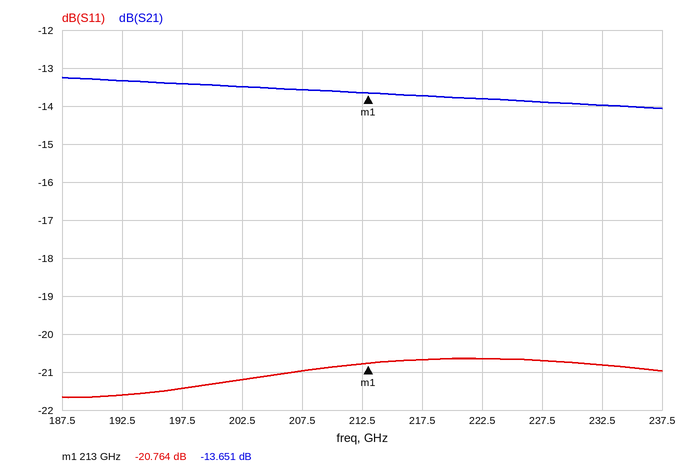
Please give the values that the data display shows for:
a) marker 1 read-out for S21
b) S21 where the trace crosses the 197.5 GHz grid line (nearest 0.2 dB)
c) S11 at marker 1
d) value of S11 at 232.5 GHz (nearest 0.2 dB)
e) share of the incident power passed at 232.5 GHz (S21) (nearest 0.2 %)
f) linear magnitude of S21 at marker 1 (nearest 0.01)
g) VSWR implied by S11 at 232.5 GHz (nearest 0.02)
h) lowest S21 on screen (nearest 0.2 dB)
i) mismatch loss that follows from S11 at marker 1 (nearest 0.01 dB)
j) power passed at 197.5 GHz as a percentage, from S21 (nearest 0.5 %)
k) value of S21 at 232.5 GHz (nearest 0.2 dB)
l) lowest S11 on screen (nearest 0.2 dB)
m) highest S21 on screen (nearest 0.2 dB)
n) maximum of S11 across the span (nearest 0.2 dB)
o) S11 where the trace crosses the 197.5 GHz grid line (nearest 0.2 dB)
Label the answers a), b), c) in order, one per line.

a) -13.651 dB
b) -13.4 dB
c) -20.764 dB
d) -20.8 dB
e) 4.0 %
f) 0.21
g) 1.20
h) -14.0 dB
i) 0.04 dB
j) 4.5 %
k) -14.0 dB
l) -21.6 dB
m) -13.2 dB
n) -20.6 dB
o) -21.4 dB
